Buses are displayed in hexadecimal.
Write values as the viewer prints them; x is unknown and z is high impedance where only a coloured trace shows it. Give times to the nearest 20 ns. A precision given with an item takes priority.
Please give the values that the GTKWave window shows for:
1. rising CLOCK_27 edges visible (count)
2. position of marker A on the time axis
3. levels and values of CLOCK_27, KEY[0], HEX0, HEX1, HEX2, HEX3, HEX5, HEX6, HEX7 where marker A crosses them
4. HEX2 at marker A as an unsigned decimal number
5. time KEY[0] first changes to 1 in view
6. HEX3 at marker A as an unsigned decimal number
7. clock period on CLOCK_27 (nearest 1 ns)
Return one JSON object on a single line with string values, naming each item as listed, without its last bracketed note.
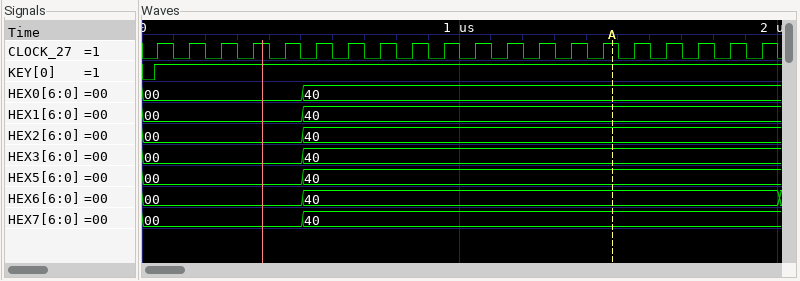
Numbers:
{"rising CLOCK_27 edges visible": "20", "position of marker A on the time axis": "1480 ns", "levels and values of CLOCK_27, KEY[0], HEX0, HEX1, HEX2, HEX3, HEX5, HEX6, HEX7 where marker A crosses them": "CLOCK_27=1, KEY[0]=1, HEX0=40, HEX1=40, HEX2=40, HEX3=40, HEX5=40, HEX6=40, HEX7=40", "HEX2 at marker A as an unsigned decimal number": "64", "time KEY[0] first changes to 1 in view": "40 ns", "HEX3 at marker A as an unsigned decimal number": "64", "clock period on CLOCK_27": "100 ns"}
